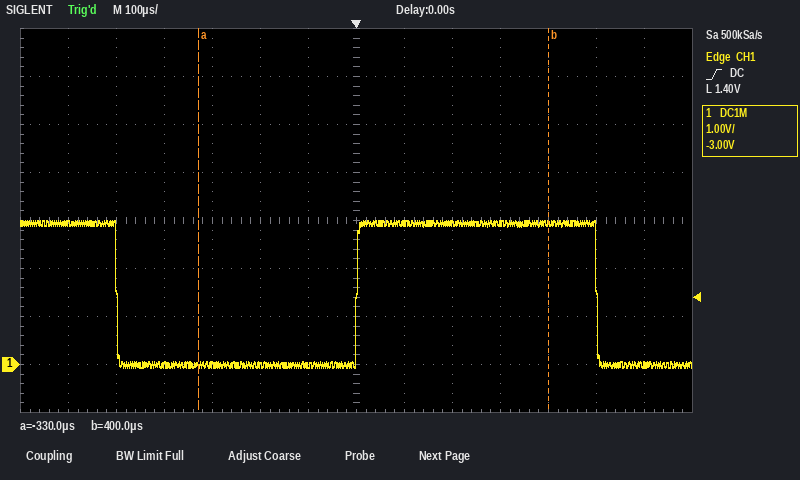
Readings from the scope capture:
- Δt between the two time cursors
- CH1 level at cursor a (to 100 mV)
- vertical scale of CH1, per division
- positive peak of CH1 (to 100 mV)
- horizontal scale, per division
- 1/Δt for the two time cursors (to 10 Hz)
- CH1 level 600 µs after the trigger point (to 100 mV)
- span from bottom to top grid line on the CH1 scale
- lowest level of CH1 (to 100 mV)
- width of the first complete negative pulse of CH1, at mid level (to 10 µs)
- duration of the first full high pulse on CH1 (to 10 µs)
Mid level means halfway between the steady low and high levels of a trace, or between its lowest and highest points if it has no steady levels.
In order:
730 µs
0.0 V
1 V
3.0 V
100 µs
1.37 kHz
0.0 V
8 V
-100 mV
500 µs
500 µs
